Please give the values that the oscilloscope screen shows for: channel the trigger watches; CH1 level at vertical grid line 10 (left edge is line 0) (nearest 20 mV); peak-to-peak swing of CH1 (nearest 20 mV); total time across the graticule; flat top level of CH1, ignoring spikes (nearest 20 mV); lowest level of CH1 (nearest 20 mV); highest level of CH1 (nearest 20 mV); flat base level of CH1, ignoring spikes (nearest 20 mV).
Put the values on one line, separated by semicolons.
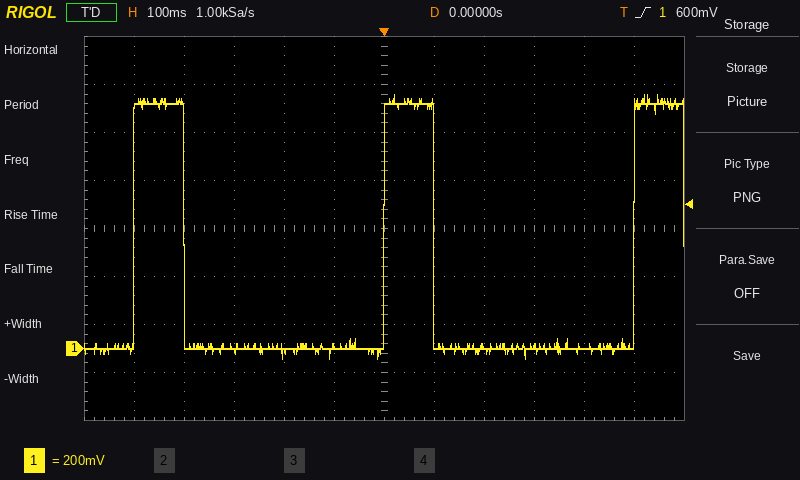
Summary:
CH1; 0 mV; 1.10 V; 1.2 s; 1.02 V; -40 mV; 1.06 V; 0 mV
